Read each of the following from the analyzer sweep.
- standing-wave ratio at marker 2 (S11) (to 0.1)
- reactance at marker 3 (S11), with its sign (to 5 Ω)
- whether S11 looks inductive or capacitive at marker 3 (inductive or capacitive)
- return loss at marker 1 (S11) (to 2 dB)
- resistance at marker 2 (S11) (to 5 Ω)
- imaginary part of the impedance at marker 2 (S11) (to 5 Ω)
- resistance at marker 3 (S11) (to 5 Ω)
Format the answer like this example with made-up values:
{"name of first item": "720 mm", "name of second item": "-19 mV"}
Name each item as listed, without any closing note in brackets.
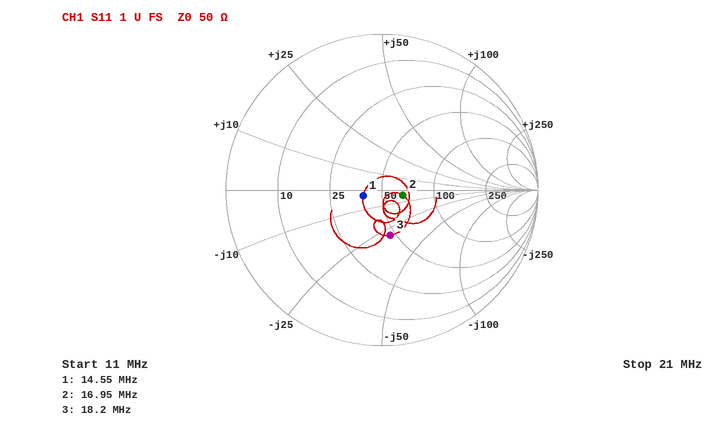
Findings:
{"standing-wave ratio at marker 2 (S11)": "1.3", "reactance at marker 3 (S11), with its sign": "-30 Ω", "whether S11 looks inductive or capacitive at marker 3": "capacitive", "return loss at marker 1 (S11)": "18 dB", "resistance at marker 2 (S11)": "65 Ω", "imaginary part of the impedance at marker 2 (S11)": "-5 Ω", "resistance at marker 3 (S11)": "45 Ω"}
